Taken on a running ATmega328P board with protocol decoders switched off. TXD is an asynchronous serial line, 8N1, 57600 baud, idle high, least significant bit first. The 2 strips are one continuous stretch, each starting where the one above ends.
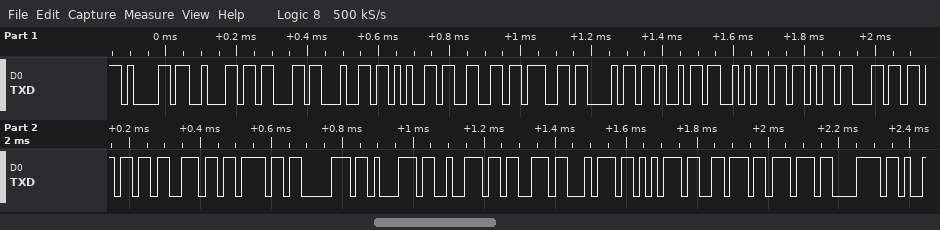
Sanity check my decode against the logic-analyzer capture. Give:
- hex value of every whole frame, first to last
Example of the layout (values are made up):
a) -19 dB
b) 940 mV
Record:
a) 0x61 0x62 0x63 0x64 0x65 0x66 0x67 0x68 0x69 0x6A 0x6B 0x6C 0x6D 0x6E 0x6F 0x70 0x71 0x72 0x73 0x74 0x75 0x76 0x77 0x78
